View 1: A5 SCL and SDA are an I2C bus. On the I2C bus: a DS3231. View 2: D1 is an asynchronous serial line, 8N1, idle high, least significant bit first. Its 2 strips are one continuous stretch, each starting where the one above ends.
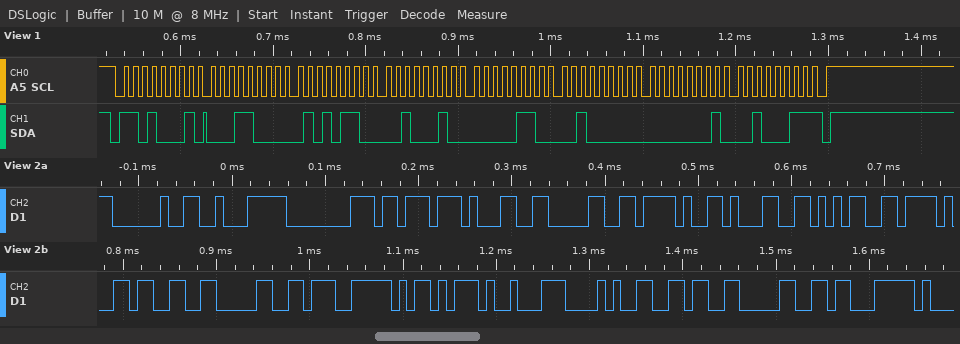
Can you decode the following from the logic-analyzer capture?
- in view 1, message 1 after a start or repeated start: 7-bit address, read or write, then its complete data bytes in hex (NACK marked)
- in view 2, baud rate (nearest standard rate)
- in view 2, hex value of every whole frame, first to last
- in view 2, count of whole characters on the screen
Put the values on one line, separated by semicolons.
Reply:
0x68 read: 18 56 22 06 20 01 23 NACK; 115200 baud; 20 E2 80 BB 31 30 2F 31 35 2F 33 30 E7 AD 89 28 36 30 E3; 19
